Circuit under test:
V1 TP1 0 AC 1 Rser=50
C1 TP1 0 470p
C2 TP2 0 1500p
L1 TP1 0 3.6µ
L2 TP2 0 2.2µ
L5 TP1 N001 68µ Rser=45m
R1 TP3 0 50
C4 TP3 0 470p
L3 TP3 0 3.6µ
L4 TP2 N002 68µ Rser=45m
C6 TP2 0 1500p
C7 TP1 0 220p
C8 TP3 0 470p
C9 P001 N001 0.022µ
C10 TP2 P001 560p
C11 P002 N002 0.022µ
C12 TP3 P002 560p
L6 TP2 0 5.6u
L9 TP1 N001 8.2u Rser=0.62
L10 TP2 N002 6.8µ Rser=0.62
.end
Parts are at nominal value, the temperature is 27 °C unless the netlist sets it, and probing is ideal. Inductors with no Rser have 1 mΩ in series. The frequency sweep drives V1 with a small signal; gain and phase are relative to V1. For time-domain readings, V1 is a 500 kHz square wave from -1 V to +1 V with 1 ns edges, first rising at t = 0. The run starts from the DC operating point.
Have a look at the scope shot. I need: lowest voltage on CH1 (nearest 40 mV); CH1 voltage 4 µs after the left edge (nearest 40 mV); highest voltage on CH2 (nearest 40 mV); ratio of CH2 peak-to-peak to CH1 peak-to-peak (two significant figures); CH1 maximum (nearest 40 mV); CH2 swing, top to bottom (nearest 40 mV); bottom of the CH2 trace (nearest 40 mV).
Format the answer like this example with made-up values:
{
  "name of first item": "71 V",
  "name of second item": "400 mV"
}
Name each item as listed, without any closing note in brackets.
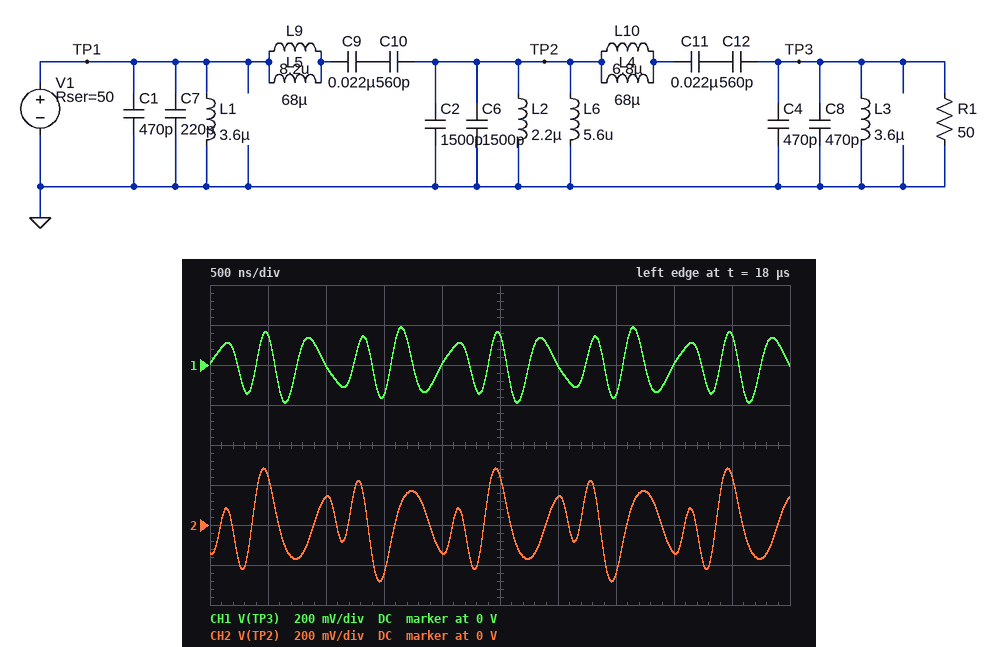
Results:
{
  "lowest voltage on CH1": "-200 mV",
  "CH1 voltage 4 µs after the left edge": "0 V",
  "highest voltage on CH2": "280 mV",
  "ratio of CH2 peak-to-peak to CH1 peak-to-peak": "1.5",
  "CH1 maximum": "200 mV",
  "CH2 swing, top to bottom": "560 mV",
  "bottom of the CH2 trace": "-280 mV"
}
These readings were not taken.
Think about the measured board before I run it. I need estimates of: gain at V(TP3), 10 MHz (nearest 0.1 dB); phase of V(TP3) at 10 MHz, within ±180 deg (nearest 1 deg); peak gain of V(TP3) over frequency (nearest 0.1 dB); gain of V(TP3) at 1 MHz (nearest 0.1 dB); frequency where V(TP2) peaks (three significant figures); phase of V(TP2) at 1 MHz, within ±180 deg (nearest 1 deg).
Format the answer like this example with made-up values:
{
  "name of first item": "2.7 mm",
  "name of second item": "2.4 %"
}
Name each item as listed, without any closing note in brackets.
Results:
{
  "gain at V(TP3), 10 MHz": "-69.8 dB",
  "phase of V(TP3) at 10 MHz, within ±180 deg": "-40 deg",
  "peak gain of V(TP3) over frequency": "-6.2 dB",
  "gain of V(TP3) at 1 MHz": "-51.4 dB",
  "frequency where V(TP2) peaks": "1.72 MHz",
  "phase of V(TP2) at 1 MHz, within ±180 deg": "-120 deg"
}
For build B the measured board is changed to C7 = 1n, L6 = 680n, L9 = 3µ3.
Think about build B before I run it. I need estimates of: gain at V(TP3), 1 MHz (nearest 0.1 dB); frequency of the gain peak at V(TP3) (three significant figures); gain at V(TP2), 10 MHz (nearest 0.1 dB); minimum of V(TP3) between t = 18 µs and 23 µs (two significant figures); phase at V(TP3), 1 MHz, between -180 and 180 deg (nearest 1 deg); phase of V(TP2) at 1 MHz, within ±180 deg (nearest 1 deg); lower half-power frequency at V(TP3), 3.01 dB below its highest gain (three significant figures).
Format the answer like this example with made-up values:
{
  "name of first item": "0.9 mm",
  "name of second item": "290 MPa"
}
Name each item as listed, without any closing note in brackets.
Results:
{
  "gain at V(TP3), 1 MHz": "-63.0 dB",
  "frequency of the gain peak at V(TP3)": "3.71 MHz",
  "gain at V(TP2), 10 MHz": "-40.5 dB",
  "minimum of V(TP3) between t = 18 µs and 23 µs": "-160 mV",
  "phase at V(TP3), 1 MHz, between -180 and 180 deg": "27 deg",
  "phase of V(TP2) at 1 MHz, within ±180 deg": "-123 deg",
  "lower half-power frequency at V(TP3), 3.01 dB below its highest gain": "3.29 MHz"
}
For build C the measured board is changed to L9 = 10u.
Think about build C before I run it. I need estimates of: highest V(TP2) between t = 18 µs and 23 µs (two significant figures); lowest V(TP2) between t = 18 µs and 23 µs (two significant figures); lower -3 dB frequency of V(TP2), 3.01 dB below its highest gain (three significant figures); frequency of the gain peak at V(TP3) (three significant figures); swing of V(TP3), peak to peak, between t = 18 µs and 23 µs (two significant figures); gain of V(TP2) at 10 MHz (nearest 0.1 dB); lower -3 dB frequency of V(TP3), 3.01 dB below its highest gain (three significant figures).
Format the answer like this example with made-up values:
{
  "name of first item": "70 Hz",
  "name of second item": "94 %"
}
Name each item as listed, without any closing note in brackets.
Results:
{
  "highest V(TP2) between t = 18 µs and 23 µs": "290 mV",
  "lowest V(TP2) between t = 18 µs and 23 µs": "-290 mV",
  "lower -3 dB frequency of V(TP2), 3.01 dB below its highest gain": "1.60 MHz",
  "frequency of the gain peak at V(TP3)": "2.37 MHz",
  "swing of V(TP3), peak to peak, between t = 18 µs and 23 µs": "350 mV",
  "gain of V(TP2) at 10 MHz": "-45.5 dB",
  "lower -3 dB frequency of V(TP3), 3.01 dB below its highest gain": "1.63 MHz"
}
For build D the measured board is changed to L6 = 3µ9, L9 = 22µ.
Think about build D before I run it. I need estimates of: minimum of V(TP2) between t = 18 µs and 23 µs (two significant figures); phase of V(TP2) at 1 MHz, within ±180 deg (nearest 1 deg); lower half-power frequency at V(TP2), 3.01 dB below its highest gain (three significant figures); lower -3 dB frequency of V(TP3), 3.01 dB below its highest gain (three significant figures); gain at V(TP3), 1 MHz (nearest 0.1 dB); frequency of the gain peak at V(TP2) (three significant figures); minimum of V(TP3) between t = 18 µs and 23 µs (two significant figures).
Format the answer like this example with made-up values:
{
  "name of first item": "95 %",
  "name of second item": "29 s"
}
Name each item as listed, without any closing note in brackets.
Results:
{
  "minimum of V(TP2) between t = 18 µs and 23 µs": "-350 mV",
  "phase of V(TP2) at 1 MHz, within ±180 deg": "-121 deg",
  "lower half-power frequency at V(TP2), 3.01 dB below its highest gain": "1.40 MHz",
  "lower -3 dB frequency of V(TP3), 3.01 dB below its highest gain": "1.87 MHz",
  "gain at V(TP3), 1 MHz": "-50.0 dB",
  "frequency of the gain peak at V(TP2)": "1.46 MHz",
  "minimum of V(TP3) between t = 18 µs and 23 µs": "-150 mV"
}
